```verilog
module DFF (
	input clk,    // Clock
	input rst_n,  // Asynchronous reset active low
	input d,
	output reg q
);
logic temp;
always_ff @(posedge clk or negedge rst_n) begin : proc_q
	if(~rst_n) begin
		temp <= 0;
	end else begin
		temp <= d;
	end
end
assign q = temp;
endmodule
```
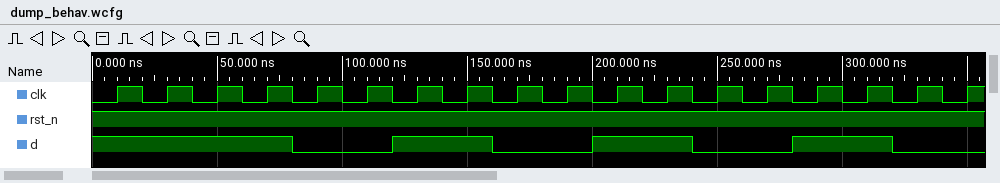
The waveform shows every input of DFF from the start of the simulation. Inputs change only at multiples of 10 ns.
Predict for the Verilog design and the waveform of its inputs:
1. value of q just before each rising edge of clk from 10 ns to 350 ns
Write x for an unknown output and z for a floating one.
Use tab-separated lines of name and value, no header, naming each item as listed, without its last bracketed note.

value of q just before each rising edge of clk from 10 ns to 350 ns	x 1 1 1 1 0 0 1 1 0 0 1 1 0 0 1 1 0
